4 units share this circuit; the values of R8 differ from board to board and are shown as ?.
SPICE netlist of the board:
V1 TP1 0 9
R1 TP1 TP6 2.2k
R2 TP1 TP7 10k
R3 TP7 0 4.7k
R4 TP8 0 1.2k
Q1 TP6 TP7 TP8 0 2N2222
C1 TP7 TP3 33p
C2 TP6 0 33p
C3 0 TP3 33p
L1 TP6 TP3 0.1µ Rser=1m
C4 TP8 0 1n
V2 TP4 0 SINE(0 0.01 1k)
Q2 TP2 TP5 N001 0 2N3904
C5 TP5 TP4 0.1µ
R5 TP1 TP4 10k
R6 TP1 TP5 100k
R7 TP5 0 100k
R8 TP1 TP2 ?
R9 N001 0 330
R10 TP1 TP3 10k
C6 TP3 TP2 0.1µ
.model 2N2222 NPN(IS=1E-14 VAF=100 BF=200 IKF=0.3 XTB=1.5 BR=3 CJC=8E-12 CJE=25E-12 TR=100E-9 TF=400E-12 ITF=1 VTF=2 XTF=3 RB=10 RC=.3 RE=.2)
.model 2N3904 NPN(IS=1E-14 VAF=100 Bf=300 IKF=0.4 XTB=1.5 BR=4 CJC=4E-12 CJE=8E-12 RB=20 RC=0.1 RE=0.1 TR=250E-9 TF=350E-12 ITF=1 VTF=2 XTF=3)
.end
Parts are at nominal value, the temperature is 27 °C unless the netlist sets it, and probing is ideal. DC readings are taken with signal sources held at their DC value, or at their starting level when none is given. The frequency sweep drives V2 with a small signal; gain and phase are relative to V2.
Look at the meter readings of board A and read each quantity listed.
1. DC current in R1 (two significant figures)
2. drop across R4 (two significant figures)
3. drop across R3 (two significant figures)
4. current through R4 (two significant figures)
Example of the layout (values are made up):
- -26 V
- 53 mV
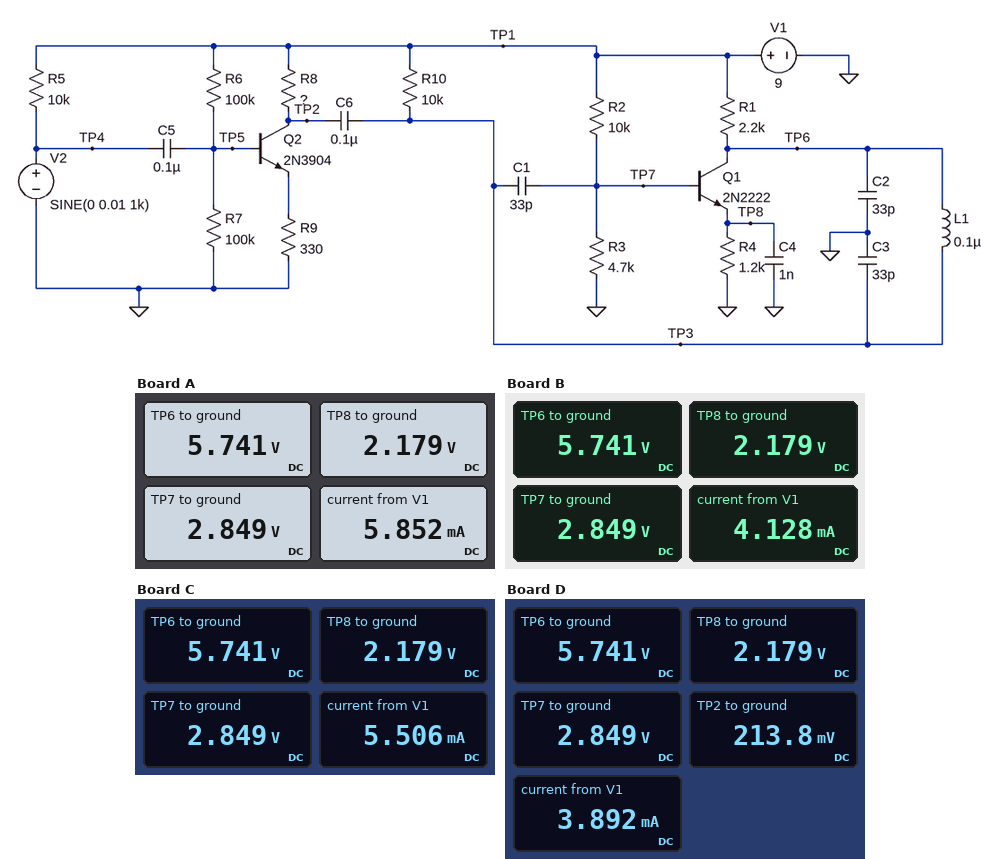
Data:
- 1.5 mA
- 2.2 V
- 2.8 V
- 1.8 mA
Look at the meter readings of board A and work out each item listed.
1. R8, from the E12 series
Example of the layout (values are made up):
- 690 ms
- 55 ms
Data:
- 3.3 kΩ
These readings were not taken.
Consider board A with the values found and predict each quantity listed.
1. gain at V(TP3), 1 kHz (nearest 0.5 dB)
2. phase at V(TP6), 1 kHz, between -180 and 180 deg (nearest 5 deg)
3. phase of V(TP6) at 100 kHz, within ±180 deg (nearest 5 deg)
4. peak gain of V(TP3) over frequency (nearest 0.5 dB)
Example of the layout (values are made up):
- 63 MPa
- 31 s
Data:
- -26.5 dB
- -70 deg
- 100 deg
- 3.5 dB
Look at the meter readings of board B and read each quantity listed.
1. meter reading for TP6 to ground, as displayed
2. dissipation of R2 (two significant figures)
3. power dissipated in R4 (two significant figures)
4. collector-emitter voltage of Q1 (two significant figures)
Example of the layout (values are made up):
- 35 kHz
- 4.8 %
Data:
- 5.741 V
- 3.8 mW
- 4.0 mW
- 3.6 V
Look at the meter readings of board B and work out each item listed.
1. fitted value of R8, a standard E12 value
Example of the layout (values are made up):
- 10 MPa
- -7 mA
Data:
- 12 kΩ
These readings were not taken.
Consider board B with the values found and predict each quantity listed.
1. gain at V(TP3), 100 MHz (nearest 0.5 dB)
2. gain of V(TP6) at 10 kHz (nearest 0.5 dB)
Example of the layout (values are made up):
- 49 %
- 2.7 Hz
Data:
- 3.0 dB
- -17.5 dB
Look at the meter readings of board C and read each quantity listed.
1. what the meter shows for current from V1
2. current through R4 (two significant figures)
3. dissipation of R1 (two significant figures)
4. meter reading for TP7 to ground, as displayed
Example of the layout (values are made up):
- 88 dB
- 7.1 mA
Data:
- 5.506 mA
- 1.8 mA
- 4.8 mW
- 2.849 V
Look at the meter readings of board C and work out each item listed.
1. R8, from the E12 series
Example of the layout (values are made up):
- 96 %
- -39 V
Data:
- 3.9 kΩ
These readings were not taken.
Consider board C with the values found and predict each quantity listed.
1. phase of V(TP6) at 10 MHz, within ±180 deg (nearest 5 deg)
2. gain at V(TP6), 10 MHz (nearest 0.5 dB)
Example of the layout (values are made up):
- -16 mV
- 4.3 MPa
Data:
- -10 deg
- -3.5 dB
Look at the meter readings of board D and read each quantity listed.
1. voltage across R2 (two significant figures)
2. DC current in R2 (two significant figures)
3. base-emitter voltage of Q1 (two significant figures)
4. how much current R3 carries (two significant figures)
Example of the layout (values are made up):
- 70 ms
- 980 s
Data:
- 6.2 V
- 620 µA
- 670 mV
- 610 µA
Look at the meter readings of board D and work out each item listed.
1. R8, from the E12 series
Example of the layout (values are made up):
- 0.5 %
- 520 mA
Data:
- 18 kΩ
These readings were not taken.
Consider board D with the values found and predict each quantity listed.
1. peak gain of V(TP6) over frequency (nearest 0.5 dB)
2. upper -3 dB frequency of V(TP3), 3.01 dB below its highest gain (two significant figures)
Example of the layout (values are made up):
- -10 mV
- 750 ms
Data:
- 12.5 dB
- 120 MHz
